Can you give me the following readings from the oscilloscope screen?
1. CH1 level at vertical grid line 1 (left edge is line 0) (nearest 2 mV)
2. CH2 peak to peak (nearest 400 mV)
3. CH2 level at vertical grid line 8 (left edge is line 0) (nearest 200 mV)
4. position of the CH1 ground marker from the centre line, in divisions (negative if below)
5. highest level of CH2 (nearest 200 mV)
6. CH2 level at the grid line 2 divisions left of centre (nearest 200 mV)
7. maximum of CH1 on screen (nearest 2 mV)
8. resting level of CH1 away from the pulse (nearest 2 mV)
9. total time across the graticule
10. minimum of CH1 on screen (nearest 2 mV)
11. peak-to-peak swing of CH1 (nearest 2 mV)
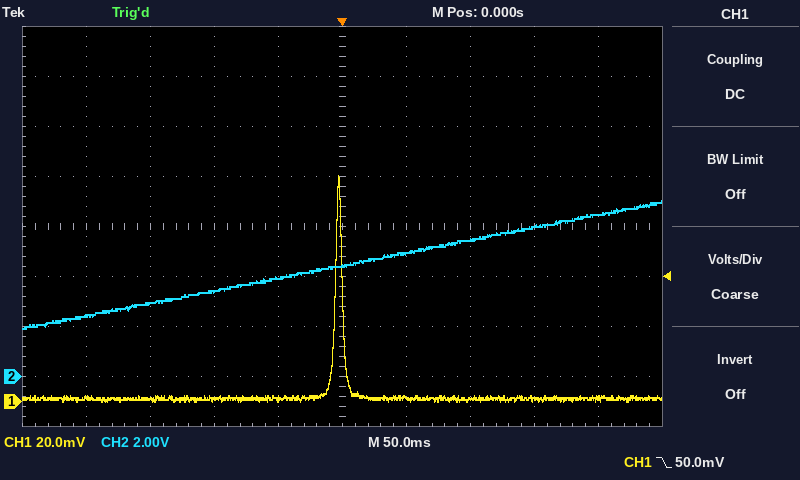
2 mV
5.2 V
6.0 V
-3.5 div
7.0 V
3.4 V
90 mV
2 mV
500 ms
0 mV
90 mV
